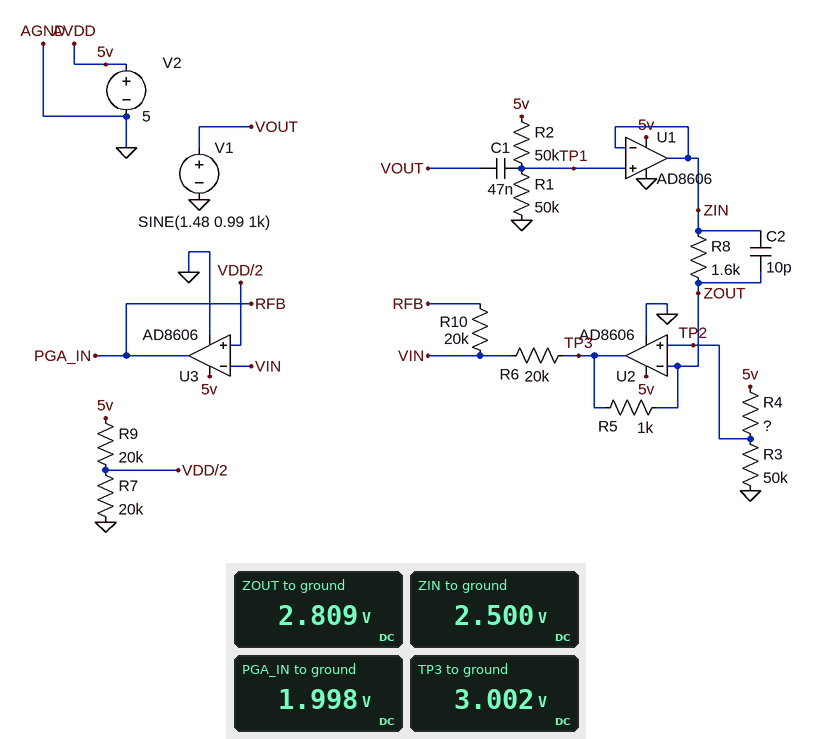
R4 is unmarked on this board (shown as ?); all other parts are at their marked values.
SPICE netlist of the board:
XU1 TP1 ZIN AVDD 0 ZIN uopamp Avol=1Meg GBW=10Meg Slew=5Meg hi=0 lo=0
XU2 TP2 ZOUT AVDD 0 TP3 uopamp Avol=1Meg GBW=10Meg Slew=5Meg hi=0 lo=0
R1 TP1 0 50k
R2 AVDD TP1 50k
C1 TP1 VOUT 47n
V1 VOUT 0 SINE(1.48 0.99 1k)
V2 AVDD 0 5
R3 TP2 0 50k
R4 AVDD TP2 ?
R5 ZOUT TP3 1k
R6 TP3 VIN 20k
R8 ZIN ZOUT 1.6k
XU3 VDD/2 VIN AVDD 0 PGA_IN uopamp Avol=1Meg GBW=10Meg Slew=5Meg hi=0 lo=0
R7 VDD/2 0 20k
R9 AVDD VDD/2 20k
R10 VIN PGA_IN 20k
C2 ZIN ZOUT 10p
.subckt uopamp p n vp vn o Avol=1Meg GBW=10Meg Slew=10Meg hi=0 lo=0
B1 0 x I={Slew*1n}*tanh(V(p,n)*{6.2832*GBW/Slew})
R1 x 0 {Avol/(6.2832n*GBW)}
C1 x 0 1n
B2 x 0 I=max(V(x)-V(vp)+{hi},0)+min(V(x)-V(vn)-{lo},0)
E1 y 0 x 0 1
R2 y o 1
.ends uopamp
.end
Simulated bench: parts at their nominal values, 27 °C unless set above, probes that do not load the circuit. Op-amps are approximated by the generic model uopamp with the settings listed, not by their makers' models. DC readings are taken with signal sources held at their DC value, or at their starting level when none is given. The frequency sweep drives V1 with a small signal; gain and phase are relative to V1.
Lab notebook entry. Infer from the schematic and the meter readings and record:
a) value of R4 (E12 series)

39 kΩ
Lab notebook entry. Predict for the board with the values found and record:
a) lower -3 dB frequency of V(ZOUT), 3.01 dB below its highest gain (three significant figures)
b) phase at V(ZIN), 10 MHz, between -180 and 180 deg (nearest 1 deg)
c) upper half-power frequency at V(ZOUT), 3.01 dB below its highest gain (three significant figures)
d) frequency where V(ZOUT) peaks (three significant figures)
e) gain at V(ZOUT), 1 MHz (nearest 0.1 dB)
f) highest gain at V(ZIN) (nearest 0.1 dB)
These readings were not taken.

5.15 MHz
-45 deg
31.0 MHz
12.6 MHz
-24.1 dB
0 dB
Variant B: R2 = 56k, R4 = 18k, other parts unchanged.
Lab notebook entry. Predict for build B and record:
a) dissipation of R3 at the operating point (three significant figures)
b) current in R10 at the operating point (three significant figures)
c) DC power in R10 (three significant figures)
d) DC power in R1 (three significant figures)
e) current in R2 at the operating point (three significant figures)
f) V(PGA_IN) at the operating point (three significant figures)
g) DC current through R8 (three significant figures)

270 µW
100 µA
200 µW
111 µW
47.2 µA
500 mV
824 µA
